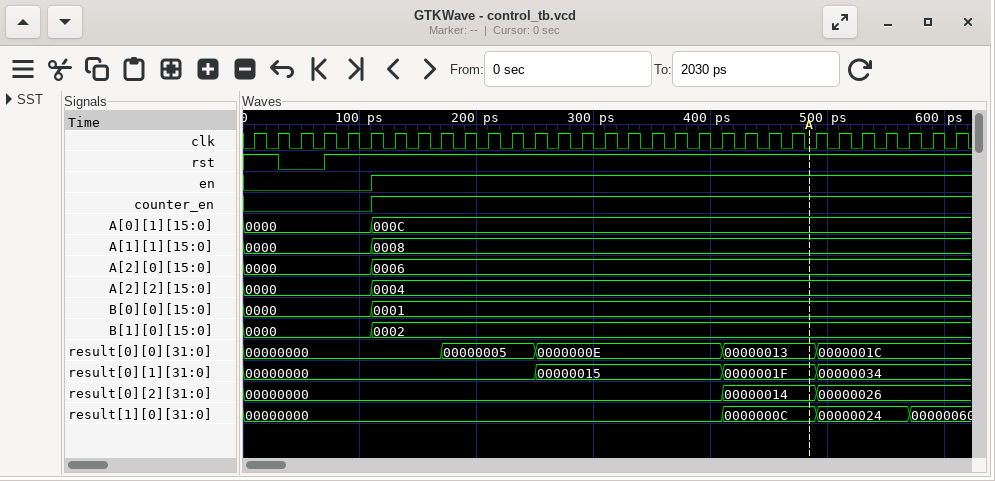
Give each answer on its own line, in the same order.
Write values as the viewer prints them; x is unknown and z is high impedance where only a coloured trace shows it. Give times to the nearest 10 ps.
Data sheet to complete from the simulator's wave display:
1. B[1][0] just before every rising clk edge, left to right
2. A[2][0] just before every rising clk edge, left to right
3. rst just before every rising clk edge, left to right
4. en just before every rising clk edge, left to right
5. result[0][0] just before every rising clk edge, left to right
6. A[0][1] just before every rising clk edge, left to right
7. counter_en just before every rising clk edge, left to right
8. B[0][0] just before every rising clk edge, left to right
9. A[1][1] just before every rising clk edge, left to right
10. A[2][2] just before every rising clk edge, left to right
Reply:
0000, 0000, 0000, 0000, 0000, 0000, 0002, 0002, 0002, 0002, 0002, 0002, 0002, 0002, 0002, 0002, 0002, 0002, 0002, 0002, 0002, 0002, 0002, 0002, 0002, 0002, 0002, 0002, 0002, 0002, 0002
0000, 0000, 0000, 0000, 0000, 0000, 0006, 0006, 0006, 0006, 0006, 0006, 0006, 0006, 0006, 0006, 0006, 0006, 0006, 0006, 0006, 0006, 0006, 0006, 0006, 0006, 0006, 0006, 0006, 0006, 0006
1 1 0 0 1 1 1 1 1 1 1 1 1 1 1 1 1 1 1 1 1 1 1 1 1 1 1 1 1 1 1
0 0 0 0 0 0 1 1 1 1 1 1 1 1 1 1 1 1 1 1 1 1 1 1 1 1 1 1 1 1 1
00000000, 00000000, 00000000, 00000000, 00000000, 00000000, 00000000, 00000000, 00000000, 00000005, 00000005, 00000005, 00000005, 0000000E, 0000000E, 0000000E, 0000000E, 0000000E, 0000000E, 0000000E, 0000000E, 00000013, 00000013, 00000013, 00000013, 0000001C, 0000001C, 0000001C, 0000001C, 0000001C, 0000001C
0000, 0000, 0000, 0000, 0000, 0000, 000C, 000C, 000C, 000C, 000C, 000C, 000C, 000C, 000C, 000C, 000C, 000C, 000C, 000C, 000C, 000C, 000C, 000C, 000C, 000C, 000C, 000C, 000C, 000C, 000C
0 0 0 0 0 0 1 1 1 1 1 1 1 1 1 1 1 1 1 1 1 1 1 1 1 1 1 1 1 1 1
0000, 0000, 0000, 0000, 0000, 0000, 0001, 0001, 0001, 0001, 0001, 0001, 0001, 0001, 0001, 0001, 0001, 0001, 0001, 0001, 0001, 0001, 0001, 0001, 0001, 0001, 0001, 0001, 0001, 0001, 0001
0000, 0000, 0000, 0000, 0000, 0000, 0008, 0008, 0008, 0008, 0008, 0008, 0008, 0008, 0008, 0008, 0008, 0008, 0008, 0008, 0008, 0008, 0008, 0008, 0008, 0008, 0008, 0008, 0008, 0008, 0008
0000, 0000, 0000, 0000, 0000, 0000, 0004, 0004, 0004, 0004, 0004, 0004, 0004, 0004, 0004, 0004, 0004, 0004, 0004, 0004, 0004, 0004, 0004, 0004, 0004, 0004, 0004, 0004, 0004, 0004, 0004
